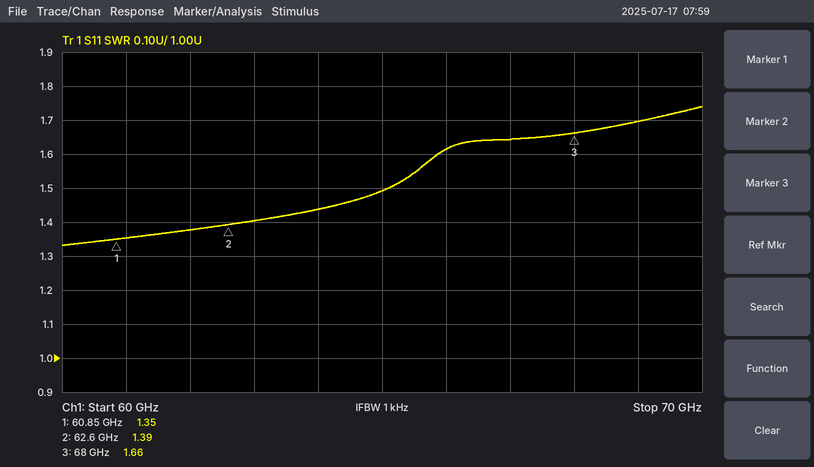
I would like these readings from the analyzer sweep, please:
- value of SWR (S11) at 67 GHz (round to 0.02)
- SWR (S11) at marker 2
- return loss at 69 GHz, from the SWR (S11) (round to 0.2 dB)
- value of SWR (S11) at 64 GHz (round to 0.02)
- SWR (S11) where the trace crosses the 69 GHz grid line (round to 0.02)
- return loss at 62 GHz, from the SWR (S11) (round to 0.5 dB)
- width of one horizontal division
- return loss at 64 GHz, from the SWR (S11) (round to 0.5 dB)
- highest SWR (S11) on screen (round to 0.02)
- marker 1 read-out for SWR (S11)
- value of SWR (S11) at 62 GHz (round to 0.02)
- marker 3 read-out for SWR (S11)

1.64
1.39
11.8 dB
1.44
1.70
16.0 dB
1 GHz
15.0 dB
1.74
1.35
1.38
1.66
